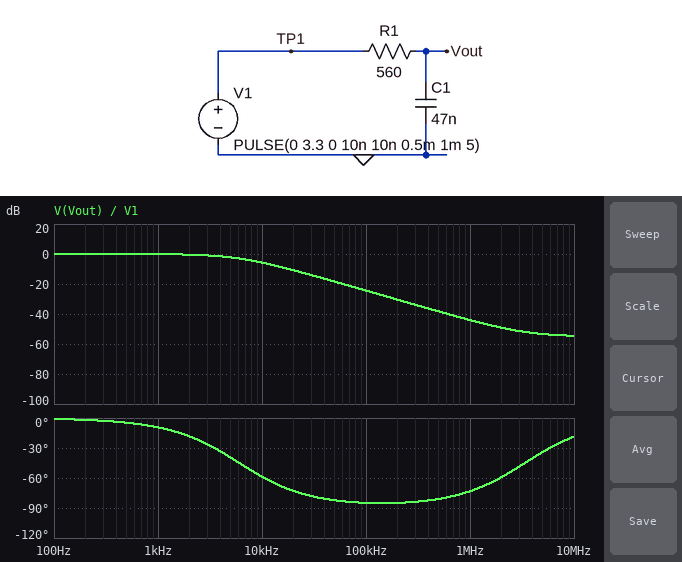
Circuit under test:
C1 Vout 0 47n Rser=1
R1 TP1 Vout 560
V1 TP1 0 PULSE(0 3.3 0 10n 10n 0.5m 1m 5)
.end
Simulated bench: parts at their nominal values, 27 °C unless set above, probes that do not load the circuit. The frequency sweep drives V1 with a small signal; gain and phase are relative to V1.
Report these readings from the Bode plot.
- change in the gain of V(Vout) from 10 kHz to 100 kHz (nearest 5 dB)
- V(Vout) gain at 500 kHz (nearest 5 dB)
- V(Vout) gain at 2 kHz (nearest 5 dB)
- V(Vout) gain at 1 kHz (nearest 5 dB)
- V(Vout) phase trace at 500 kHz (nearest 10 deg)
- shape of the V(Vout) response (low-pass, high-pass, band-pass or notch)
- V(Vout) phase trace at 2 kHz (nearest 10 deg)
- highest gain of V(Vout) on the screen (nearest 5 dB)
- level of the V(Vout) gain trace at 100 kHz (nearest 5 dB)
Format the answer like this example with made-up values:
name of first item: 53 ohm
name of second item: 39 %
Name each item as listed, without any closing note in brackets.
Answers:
change in the gain of V(Vout) from 10 kHz to 100 kHz: -20 dB
V(Vout) gain at 500 kHz: -40 dB
V(Vout) gain at 2 kHz: 0 dB
V(Vout) gain at 1 kHz: 0 dB
V(Vout) phase trace at 500 kHz: -80 deg
shape of the V(Vout) response: low-pass
V(Vout) phase trace at 2 kHz: -20 deg
highest gain of V(Vout) on the screen: 0 dB
level of the V(Vout) gain trace at 100 kHz: -25 dB
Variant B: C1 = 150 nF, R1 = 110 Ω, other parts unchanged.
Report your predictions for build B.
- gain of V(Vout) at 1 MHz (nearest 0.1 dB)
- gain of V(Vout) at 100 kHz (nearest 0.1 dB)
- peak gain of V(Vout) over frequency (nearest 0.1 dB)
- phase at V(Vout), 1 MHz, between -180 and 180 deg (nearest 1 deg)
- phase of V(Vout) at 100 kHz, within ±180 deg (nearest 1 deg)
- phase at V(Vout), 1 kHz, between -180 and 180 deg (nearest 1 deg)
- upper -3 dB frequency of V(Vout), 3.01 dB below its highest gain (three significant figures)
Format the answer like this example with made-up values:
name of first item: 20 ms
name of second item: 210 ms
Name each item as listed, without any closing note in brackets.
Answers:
gain of V(Vout) at 1 MHz: -37.6 dB
gain of V(Vout) at 100 kHz: -20.4 dB
peak gain of V(Vout) over frequency: 0 dB
phase at V(Vout), 1 MHz, between -180 and 180 deg: -46 deg
phase of V(Vout) at 100 kHz, within ±180 deg: -79 deg
phase at V(Vout), 1 kHz, between -180 and 180 deg: -6 deg
upper -3 dB frequency of V(Vout), 3.01 dB below its highest gain: 9.56 kHz
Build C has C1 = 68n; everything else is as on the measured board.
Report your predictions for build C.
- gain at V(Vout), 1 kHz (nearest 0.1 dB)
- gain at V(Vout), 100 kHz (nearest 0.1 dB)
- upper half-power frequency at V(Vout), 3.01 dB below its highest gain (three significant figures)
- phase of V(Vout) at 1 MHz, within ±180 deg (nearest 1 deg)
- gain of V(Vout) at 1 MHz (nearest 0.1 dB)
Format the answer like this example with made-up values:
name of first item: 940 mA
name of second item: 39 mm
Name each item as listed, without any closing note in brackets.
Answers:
gain at V(Vout), 1 kHz: -0.2 dB
gain at V(Vout), 100 kHz: -27.6 dB
upper half-power frequency at V(Vout), 3.01 dB below its highest gain: 4.17 kHz
phase of V(Vout) at 1 MHz, within ±180 deg: -67 deg
gain of V(Vout) at 1 MHz: -46.9 dB
